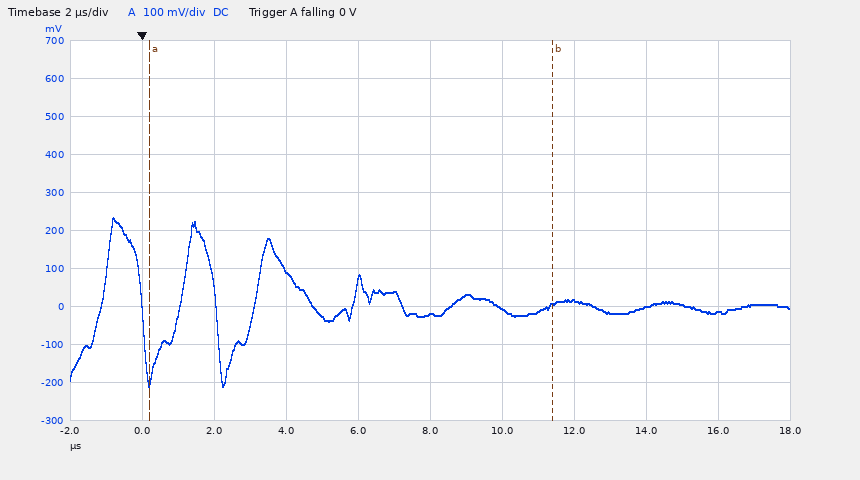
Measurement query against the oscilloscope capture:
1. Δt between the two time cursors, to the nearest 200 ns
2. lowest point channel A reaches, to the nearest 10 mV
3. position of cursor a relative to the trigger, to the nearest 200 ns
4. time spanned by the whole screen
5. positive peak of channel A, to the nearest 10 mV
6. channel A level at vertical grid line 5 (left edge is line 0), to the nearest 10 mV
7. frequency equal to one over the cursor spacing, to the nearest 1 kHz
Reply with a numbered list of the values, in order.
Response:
1. 11.2 µs
2. -210 mV
3. +200 ns
4. 20 µs
5. 230 mV
6. -20 mV
7. 89 kHz
